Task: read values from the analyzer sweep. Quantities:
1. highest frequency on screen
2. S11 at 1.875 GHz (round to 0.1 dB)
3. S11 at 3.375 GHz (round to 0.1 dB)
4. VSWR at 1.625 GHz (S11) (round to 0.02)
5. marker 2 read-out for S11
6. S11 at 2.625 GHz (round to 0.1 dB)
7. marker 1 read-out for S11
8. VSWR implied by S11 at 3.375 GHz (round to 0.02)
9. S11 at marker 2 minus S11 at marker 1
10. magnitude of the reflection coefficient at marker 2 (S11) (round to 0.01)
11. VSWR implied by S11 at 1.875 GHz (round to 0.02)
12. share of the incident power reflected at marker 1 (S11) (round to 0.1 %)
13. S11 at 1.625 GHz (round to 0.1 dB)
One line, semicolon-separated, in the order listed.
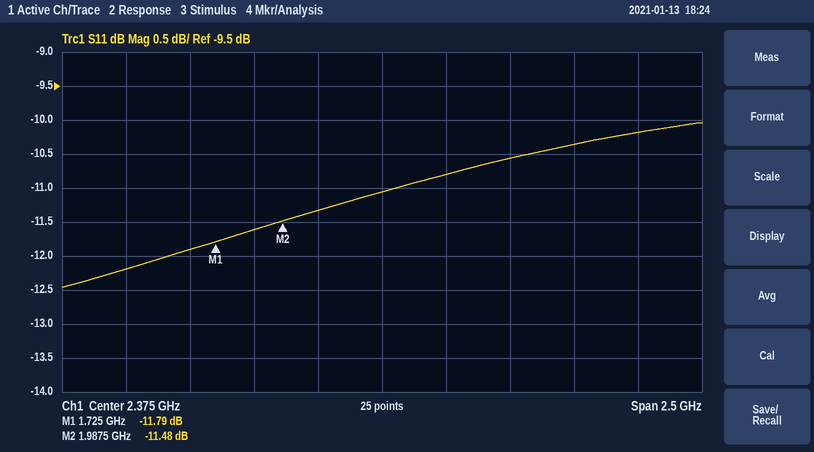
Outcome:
3.625 GHz; -11.6 dB; -10.2 dB; 1.68; -11.48 dB; -10.8 dB; -11.79 dB; 1.90; 0.31 dB; 0.27; 1.72; 6.6 %; -11.9 dB
